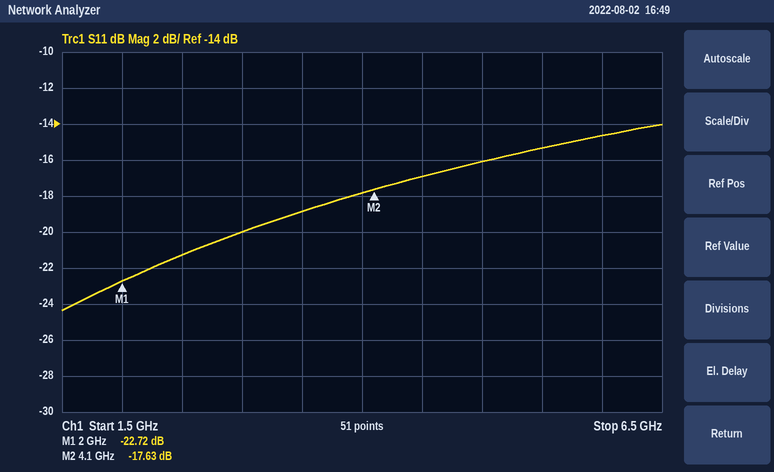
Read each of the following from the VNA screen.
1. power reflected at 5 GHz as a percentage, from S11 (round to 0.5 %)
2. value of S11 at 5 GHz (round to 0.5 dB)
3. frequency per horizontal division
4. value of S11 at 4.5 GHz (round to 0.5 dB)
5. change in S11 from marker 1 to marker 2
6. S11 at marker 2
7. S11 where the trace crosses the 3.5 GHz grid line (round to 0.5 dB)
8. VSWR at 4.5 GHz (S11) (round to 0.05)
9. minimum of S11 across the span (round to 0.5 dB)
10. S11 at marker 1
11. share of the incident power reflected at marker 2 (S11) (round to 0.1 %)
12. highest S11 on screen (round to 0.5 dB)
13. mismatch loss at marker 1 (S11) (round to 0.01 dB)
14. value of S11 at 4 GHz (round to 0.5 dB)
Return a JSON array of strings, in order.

["2.5 %", "-16.0 dB", "500 MHz", "-17.0 dB", "5.09 dB", "-17.63 dB", "-19.0 dB", "1.35", "-24.5 dB", "-22.72 dB", "1.7 %", "-14.0 dB", "0.02 dB", "-18.0 dB"]
